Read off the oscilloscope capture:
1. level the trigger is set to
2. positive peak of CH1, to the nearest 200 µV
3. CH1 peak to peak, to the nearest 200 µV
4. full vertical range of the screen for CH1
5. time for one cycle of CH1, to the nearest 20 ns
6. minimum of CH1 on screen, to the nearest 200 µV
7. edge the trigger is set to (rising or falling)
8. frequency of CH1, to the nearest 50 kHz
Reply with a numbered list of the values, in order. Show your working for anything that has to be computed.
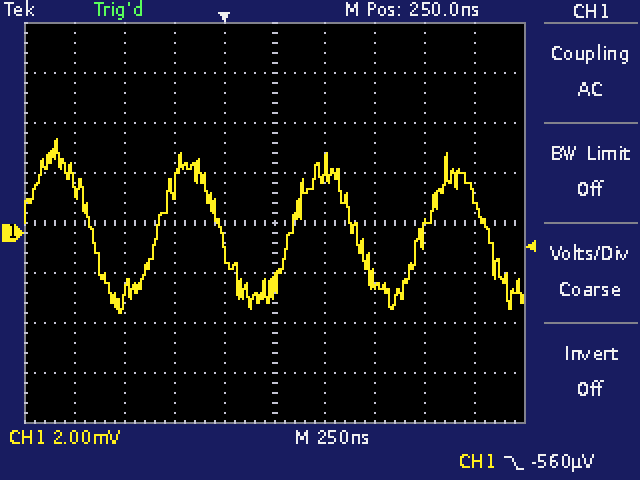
1. -560 µV
2. 3.8 mV
3. 3.8 mV − (-3.2 mV) = 7.0 mV
4. 16 mV
5. 660 ns
6. -3.2 mV
7. falling
8. 1 / 660 ns ≈ 1.52 MHz, so 1.50 MHz to the nearest 50 kHz
